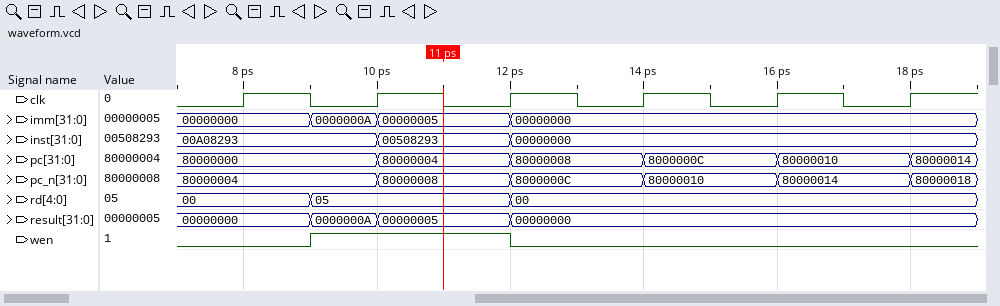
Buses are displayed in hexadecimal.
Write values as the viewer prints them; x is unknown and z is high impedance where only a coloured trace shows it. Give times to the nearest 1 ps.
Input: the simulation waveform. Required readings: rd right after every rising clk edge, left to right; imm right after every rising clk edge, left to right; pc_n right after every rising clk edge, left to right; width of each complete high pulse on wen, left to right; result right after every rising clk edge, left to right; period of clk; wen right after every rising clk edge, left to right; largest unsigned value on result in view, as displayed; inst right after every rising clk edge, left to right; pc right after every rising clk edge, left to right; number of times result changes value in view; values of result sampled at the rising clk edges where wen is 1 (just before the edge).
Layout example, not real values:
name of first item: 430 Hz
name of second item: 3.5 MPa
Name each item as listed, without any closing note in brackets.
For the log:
rd right after every rising clk edge, left to right: 00, 05, 00, 00, 00, 00
imm right after every rising clk edge, left to right: 00000000, 00000005, 00000000, 00000000, 00000000, 00000000
pc_n right after every rising clk edge, left to right: 80000004, 80000008, 8000000C, 80000010, 80000014, 80000018
width of each complete high pulse on wen, left to right: 3 ps
result right after every rising clk edge, left to right: 00000000, 00000005, 00000000, 00000000, 00000000, 00000000
period of clk: 2 ps
wen right after every rising clk edge, left to right: 0 1 0 0 0 0
largest unsigned value on result in view, as displayed: 0000000A
inst right after every rising clk edge, left to right: 00A08293, 00508293, 00000000, 00000000, 00000000, 00000000
pc right after every rising clk edge, left to right: 80000000, 80000004, 80000008, 8000000C, 80000010, 80000014
number of times result changes value in view: 3
values of result sampled at the rising clk edges where wen is 1: 0000000A, 00000005
